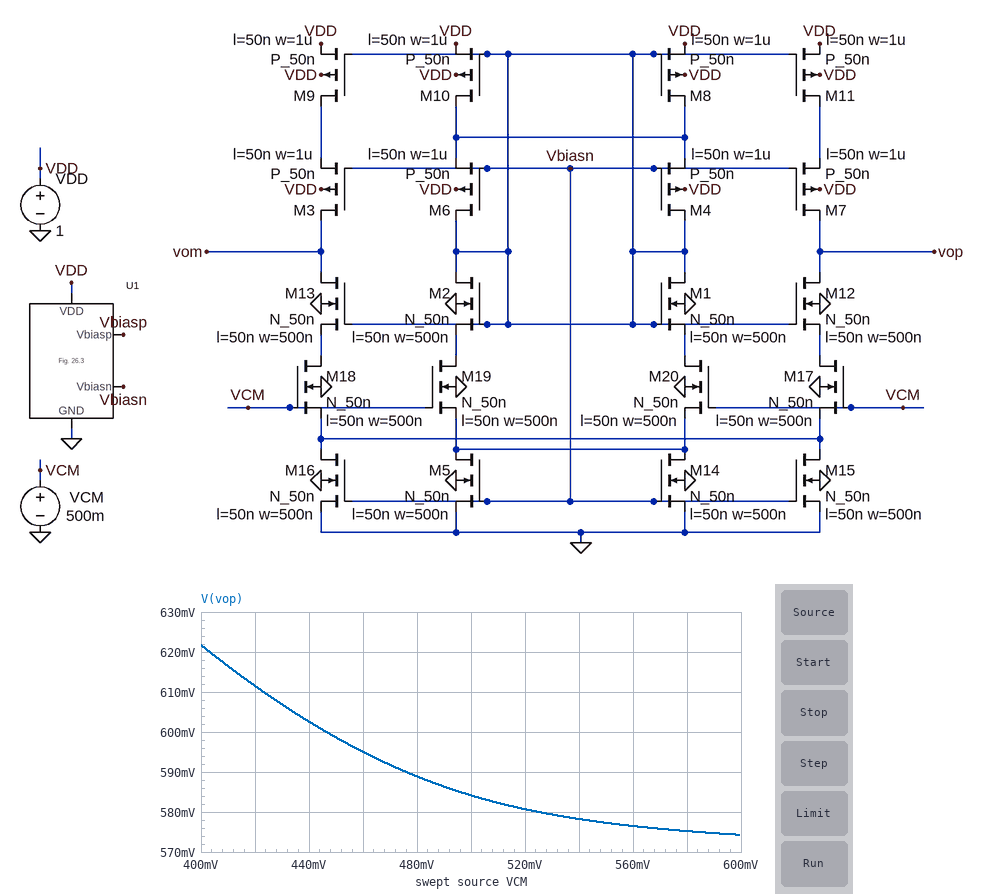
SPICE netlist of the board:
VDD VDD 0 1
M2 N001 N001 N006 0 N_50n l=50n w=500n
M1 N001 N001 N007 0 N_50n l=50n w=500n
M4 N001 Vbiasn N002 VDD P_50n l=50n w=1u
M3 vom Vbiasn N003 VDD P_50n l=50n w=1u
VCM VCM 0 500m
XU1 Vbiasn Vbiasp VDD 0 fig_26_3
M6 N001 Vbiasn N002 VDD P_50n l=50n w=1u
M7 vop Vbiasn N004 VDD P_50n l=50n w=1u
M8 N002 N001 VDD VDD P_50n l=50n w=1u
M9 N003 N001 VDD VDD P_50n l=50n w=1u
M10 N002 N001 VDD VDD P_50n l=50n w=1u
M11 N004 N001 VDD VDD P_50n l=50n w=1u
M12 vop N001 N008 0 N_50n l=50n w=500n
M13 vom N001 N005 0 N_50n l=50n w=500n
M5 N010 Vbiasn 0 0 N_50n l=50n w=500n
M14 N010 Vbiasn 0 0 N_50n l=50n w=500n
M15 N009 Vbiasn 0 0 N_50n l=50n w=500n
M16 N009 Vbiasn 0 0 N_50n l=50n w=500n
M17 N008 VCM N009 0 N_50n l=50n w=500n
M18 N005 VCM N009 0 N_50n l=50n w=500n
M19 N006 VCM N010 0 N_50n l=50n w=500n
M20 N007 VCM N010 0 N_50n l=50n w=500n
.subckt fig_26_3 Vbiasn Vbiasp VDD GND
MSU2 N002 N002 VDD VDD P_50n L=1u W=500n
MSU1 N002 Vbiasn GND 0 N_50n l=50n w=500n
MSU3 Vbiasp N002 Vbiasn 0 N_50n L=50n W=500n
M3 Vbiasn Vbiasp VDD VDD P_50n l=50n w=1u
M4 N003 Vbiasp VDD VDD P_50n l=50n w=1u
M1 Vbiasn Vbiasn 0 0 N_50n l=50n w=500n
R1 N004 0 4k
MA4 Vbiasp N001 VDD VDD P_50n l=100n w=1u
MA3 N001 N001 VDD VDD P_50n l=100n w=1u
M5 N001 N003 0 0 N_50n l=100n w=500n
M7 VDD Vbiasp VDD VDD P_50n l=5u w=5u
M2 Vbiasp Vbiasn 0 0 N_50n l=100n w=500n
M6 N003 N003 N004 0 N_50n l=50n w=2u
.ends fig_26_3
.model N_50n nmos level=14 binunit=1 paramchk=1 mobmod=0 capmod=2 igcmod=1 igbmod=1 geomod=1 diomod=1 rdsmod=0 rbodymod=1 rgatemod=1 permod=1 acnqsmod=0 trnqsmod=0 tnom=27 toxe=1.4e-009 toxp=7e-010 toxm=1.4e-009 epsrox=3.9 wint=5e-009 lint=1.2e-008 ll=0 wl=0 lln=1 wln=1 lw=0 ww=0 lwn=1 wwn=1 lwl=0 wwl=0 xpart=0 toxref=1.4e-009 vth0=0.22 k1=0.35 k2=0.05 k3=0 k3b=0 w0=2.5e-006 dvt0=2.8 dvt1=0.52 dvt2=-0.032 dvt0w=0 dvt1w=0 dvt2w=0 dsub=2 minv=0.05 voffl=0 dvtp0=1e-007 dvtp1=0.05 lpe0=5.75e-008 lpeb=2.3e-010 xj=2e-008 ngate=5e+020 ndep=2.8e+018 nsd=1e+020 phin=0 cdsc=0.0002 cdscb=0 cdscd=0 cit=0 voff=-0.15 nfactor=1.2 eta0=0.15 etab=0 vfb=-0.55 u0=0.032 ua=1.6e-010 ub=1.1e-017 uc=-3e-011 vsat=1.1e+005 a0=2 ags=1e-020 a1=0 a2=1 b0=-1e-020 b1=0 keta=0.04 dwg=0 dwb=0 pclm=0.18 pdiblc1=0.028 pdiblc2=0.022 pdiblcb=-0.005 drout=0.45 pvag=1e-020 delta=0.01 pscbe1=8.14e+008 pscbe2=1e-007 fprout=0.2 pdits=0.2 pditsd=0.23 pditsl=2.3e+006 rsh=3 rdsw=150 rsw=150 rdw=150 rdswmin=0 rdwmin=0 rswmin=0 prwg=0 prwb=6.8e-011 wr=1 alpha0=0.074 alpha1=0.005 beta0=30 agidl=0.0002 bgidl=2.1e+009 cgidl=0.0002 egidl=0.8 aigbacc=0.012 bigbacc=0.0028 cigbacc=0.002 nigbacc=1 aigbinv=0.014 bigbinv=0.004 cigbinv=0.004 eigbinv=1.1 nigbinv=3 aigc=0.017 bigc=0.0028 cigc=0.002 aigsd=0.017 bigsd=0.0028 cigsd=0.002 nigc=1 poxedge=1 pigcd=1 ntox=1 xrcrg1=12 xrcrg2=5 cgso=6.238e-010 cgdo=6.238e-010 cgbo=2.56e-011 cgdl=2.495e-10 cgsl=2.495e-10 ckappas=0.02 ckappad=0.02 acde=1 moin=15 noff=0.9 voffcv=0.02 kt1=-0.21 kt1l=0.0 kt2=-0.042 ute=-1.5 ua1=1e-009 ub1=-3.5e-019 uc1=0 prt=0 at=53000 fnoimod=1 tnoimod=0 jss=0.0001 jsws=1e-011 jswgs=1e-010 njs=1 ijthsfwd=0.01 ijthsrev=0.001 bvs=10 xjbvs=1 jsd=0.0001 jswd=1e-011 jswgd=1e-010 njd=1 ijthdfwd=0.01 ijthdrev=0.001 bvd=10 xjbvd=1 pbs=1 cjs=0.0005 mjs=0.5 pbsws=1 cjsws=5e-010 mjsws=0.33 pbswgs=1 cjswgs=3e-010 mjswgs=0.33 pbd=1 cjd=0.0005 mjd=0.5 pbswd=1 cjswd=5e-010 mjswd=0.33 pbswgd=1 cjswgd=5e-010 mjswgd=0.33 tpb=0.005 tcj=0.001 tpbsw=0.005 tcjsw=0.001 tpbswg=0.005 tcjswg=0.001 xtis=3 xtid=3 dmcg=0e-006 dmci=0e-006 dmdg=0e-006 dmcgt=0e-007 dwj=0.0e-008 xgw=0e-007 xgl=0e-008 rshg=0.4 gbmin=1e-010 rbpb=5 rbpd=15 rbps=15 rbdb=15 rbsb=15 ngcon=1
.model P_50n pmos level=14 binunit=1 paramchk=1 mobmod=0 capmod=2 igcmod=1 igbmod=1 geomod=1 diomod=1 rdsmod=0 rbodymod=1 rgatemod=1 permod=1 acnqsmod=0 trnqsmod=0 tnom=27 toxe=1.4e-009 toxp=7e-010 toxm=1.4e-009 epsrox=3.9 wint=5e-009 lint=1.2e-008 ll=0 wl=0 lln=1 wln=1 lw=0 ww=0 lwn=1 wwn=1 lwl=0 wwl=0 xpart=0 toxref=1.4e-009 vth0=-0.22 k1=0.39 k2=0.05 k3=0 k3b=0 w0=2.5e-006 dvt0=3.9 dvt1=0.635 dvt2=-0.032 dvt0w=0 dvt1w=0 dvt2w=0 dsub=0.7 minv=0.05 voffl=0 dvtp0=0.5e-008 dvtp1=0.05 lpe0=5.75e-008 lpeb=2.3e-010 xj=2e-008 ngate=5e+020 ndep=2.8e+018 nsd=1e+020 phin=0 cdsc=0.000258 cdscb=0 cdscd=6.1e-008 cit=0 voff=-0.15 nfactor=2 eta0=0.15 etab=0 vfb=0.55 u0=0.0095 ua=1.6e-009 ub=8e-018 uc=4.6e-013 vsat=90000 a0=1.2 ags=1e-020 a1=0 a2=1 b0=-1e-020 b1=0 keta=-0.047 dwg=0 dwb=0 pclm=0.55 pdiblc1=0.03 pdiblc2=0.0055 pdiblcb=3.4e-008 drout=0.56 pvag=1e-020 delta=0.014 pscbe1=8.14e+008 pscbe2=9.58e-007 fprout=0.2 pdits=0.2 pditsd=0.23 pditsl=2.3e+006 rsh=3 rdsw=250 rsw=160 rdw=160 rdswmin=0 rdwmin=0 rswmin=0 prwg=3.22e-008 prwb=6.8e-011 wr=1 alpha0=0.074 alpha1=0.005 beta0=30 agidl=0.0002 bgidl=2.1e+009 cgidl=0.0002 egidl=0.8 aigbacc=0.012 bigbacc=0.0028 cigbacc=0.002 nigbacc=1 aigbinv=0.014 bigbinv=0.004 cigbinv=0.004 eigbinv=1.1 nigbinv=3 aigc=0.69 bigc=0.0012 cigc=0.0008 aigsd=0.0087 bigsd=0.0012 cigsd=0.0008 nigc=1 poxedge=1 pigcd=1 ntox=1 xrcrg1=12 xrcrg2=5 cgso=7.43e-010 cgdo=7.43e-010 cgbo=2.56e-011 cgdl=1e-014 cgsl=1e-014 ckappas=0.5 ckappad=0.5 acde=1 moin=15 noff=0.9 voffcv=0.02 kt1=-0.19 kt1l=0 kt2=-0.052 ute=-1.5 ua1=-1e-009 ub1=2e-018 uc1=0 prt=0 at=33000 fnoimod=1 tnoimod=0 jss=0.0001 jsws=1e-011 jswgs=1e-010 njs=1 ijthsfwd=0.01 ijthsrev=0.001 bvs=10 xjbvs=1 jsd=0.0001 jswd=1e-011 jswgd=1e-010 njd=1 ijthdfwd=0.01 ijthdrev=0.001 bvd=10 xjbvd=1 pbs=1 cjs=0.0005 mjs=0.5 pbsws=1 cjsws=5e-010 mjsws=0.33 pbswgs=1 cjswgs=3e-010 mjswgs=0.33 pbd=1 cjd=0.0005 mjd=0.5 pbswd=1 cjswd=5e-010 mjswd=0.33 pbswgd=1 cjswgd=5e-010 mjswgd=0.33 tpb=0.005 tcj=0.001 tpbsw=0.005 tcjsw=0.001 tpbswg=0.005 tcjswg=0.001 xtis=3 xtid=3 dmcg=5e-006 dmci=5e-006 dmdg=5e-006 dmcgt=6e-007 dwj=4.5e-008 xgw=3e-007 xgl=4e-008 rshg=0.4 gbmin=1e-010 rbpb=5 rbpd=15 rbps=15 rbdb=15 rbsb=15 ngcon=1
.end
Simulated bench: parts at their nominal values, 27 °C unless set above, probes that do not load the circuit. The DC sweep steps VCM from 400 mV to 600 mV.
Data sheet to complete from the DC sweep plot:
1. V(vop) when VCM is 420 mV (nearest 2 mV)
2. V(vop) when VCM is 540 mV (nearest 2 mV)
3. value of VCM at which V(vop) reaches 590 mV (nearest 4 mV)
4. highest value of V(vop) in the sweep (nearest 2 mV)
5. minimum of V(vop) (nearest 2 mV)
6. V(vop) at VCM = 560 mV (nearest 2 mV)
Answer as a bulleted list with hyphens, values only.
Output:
- 612 mV
- 578 mV
- 476 mV
- 622 mV
- 574 mV
- 576 mV
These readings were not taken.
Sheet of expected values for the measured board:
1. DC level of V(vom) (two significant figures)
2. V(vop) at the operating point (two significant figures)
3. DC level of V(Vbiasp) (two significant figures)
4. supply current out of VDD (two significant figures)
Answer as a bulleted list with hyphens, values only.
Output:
- 580 mV
- 580 mV
- 590 mV
- 110 µA
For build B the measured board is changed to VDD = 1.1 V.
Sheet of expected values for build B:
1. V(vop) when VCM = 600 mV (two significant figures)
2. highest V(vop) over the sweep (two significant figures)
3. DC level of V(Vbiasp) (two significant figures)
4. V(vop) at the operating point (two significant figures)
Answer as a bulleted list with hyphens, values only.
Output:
- 680 mV
- 730 mV
- 700 mV
- 690 mV
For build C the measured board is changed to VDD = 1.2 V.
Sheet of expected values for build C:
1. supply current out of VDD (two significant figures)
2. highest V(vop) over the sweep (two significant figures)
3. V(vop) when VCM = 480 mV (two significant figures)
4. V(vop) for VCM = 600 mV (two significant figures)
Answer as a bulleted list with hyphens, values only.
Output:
- 120 µA
- 830 mV
- 800 mV
- 780 mV
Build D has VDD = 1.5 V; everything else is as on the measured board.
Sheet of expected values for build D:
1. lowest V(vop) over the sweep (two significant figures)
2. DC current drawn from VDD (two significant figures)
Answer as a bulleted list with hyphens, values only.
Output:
- 1.1 V
- 130 µA
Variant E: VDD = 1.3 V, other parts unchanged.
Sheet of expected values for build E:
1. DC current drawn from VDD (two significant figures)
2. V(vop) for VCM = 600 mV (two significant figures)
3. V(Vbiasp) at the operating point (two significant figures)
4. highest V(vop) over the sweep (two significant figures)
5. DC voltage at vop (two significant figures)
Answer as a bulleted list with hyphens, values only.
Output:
- 120 µA
- 890 mV
- 910 mV
- 930 mV
- 900 mV
